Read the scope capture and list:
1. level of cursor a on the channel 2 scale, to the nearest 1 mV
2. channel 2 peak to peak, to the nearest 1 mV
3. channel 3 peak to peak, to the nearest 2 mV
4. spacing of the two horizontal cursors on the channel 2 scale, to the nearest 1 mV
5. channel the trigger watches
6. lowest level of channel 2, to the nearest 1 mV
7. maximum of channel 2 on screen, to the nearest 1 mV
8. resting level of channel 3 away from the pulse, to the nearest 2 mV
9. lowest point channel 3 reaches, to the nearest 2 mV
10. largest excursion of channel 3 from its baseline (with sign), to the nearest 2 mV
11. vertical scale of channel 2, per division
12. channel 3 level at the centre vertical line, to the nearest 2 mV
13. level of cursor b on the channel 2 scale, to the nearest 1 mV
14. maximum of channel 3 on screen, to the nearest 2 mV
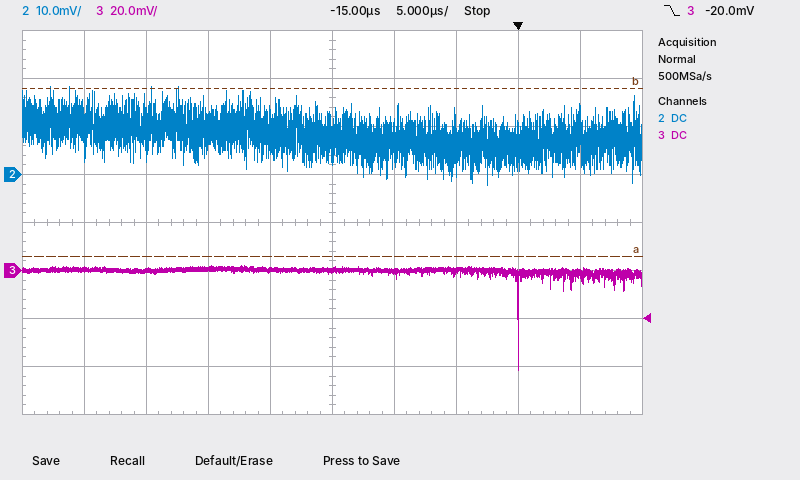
-17 mV
20 mV
44 mV
35 mV
channel 3
-2 mV
18 mV
0 mV
-42 mV
-42 mV
10 mV
0 mV
18 mV
2 mV
